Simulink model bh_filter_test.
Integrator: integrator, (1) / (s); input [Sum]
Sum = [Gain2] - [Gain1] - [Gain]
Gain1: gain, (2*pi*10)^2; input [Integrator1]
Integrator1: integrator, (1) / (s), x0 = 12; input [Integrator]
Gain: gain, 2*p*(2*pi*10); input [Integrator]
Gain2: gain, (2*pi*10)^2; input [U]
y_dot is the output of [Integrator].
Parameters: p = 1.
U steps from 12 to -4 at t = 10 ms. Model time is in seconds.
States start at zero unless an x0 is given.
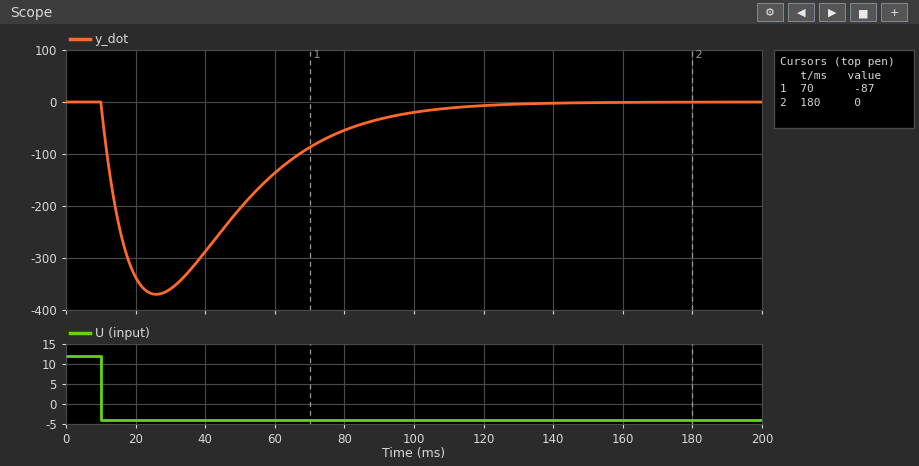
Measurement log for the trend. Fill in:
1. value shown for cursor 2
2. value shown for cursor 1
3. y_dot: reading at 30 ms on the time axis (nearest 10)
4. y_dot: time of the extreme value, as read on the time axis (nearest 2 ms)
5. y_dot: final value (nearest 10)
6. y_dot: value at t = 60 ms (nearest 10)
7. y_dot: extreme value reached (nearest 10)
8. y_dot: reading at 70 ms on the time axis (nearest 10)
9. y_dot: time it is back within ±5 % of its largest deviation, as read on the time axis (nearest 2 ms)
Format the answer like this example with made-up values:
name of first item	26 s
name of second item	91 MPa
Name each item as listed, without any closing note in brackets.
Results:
value shown for cursor 2	0
value shown for cursor 1	-87
y_dot: reading at 30 ms on the time axis	-360
y_dot: time of the extreme value, as read on the time axis	26 ms
y_dot: final value	0
y_dot: value at t = 60 ms	-140
y_dot: extreme value reached	-370
y_dot: reading at 70 ms on the time axis	-90
y_dot: time it is back within ±5 % of its largest deviation, as read on the time axis	102 ms
